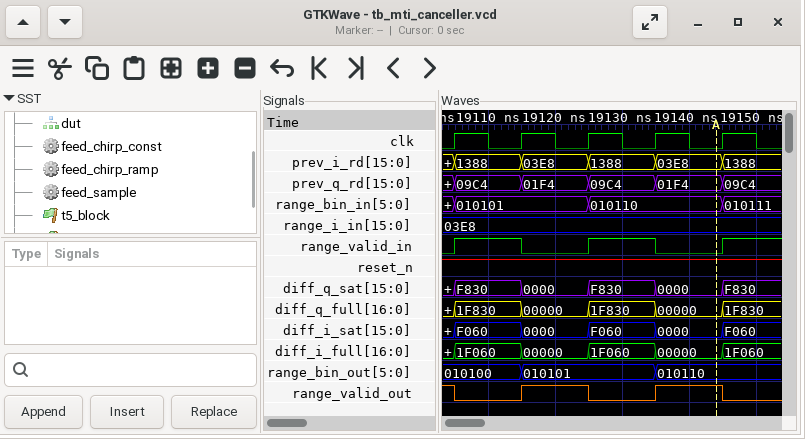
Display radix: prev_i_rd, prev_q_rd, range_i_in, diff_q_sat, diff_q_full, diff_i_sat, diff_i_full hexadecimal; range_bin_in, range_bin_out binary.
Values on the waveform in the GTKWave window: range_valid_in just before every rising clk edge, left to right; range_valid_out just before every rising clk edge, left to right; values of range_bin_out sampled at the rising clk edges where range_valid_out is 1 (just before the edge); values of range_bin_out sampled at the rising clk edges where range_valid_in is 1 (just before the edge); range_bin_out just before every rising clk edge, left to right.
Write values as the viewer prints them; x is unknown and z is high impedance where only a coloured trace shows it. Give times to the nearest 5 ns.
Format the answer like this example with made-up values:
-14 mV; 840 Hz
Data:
0 1 0 1 0; 1 0 1 0 1; 010100, 010101, 010110; 010100, 010101; 010100, 010100, 010101, 010101, 010110
